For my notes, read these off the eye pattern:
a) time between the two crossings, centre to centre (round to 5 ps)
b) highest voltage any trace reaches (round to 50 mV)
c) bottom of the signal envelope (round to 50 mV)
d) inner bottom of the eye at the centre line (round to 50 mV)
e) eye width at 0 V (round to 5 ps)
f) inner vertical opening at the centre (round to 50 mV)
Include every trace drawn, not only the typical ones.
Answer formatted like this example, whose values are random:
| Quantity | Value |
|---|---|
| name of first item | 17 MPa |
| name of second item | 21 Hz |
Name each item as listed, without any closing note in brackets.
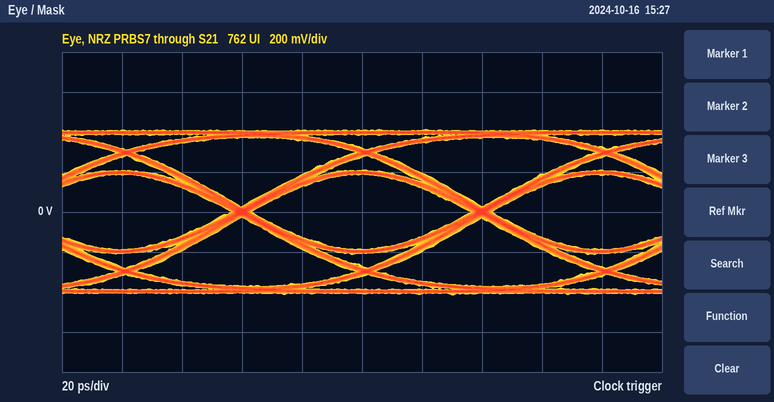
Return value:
| Quantity | Value |
|---|---|
| time between the two crossings, centre to centre | 80 ps |
| highest voltage any trace reaches | 400 mV |
| bottom of the signal envelope | -400 mV |
| inner bottom of the eye at the centre line | -200 mV |
| eye width at 0 V | 75 ps |
| inner vertical opening at the centre | 400 mV |
